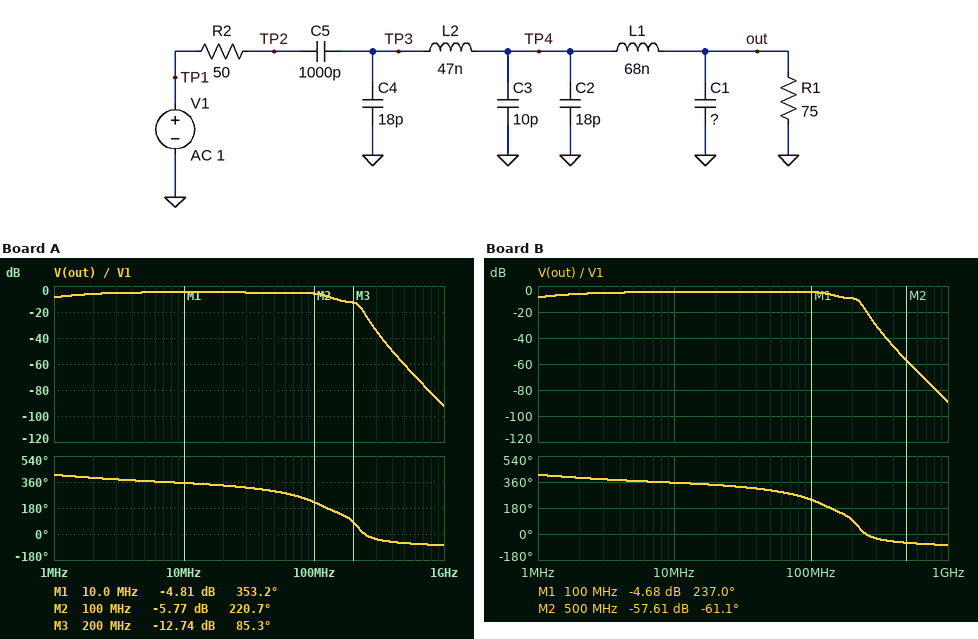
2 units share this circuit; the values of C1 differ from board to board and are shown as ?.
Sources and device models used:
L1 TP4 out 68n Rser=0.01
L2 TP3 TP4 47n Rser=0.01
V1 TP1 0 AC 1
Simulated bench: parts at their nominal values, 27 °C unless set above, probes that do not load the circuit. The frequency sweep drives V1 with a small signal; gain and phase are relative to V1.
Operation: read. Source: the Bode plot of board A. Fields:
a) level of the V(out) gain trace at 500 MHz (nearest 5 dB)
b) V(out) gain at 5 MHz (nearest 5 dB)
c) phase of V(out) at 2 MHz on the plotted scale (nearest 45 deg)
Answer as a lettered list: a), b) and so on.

a) -60 dB
b) -5 dB
c) 405 deg
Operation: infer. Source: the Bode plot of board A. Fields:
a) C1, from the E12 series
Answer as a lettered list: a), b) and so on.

a) 56 pF
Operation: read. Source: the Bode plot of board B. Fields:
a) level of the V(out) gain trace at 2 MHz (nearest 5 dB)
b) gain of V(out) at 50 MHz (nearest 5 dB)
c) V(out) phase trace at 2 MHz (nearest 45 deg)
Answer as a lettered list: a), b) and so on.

a) -5 dB
b) -5 dB
c) 405 deg
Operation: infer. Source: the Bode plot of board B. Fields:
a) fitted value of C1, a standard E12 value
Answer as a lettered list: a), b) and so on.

a) 39 pF
